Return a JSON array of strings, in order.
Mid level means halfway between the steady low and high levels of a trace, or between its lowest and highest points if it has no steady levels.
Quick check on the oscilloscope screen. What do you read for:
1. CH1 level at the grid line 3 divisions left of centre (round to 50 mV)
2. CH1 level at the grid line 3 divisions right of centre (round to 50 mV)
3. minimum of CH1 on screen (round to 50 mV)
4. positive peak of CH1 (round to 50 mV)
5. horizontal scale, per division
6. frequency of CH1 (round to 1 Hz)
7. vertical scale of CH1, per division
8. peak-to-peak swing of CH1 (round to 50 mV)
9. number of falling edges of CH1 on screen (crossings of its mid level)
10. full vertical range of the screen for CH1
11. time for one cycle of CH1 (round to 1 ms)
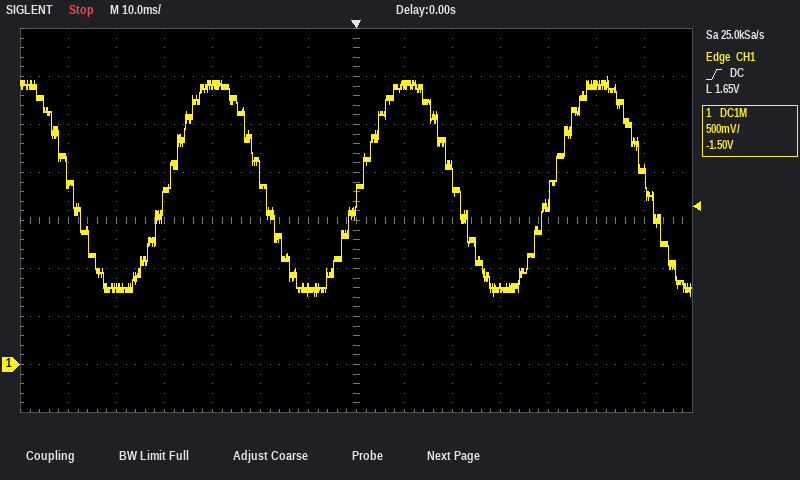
["2.90 V", "800 mV", "700 mV", "3.00 V", "10 ms", "25 Hz", "500 mV", "2.30 V", "4", "4 V", "40 ms"]
